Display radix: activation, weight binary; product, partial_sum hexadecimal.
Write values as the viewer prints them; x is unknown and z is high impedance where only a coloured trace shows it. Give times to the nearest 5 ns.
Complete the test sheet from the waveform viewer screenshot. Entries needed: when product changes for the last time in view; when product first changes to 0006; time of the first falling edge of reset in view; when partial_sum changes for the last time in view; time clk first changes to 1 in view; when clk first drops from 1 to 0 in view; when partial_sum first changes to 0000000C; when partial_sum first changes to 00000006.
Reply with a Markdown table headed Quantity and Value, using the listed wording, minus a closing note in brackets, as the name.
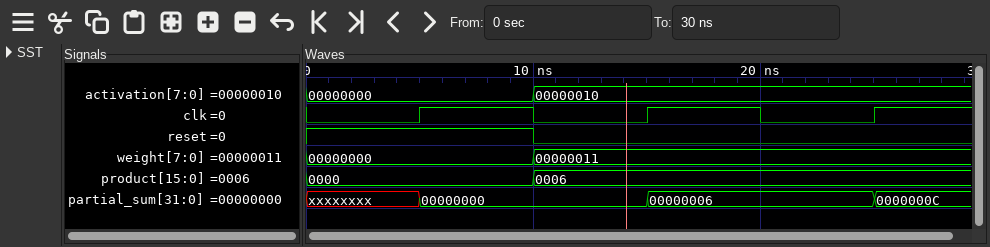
| Quantity | Value |
|---|---|
| when product changes for the last time in view | 10 ns |
| when product first changes to 0006 | 10 ns |
| time of the first falling edge of reset in view | 10 ns |
| when partial_sum changes for the last time in view | 25 ns |
| time clk first changes to 1 in view | 5 ns |
| when clk first drops from 1 to 0 in view | 10 ns |
| when partial_sum first changes to 0000000C | 25 ns |
| when partial_sum first changes to 00000006 | 15 ns |
